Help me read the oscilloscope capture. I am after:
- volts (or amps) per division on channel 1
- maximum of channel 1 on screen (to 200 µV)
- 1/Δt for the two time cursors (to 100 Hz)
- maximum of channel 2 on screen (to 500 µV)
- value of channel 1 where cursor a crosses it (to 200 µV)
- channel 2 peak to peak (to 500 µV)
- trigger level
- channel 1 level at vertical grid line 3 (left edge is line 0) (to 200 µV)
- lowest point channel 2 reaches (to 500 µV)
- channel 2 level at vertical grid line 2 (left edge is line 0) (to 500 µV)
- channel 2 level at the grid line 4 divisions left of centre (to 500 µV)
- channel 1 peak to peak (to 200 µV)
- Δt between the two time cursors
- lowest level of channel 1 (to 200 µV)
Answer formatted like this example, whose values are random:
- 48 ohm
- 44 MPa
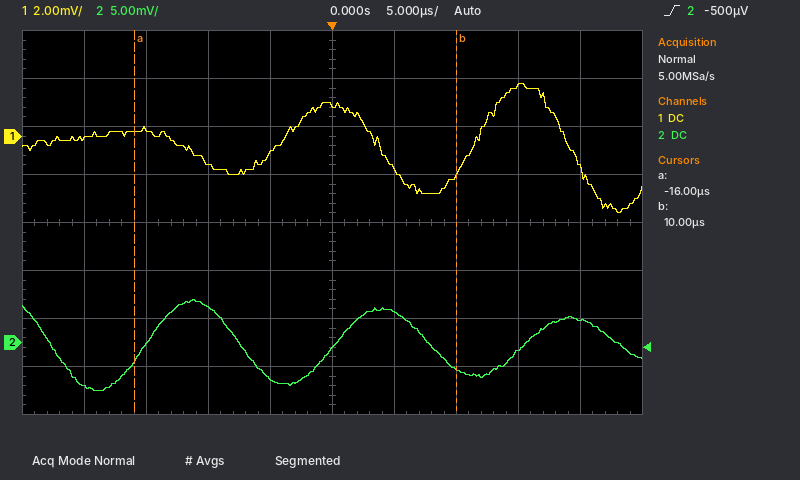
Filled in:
- 2 mV
- 2.2 mV
- 38.5 kHz
- 4.5 mV
- 200 µV
- 9.5 mV
- -500 µV
- -1.2 mV
- -5.0 mV
- 0.0 mV
- -4.5 mV
- 5.4 mV
- 26.0 µs
- -3.2 mV
